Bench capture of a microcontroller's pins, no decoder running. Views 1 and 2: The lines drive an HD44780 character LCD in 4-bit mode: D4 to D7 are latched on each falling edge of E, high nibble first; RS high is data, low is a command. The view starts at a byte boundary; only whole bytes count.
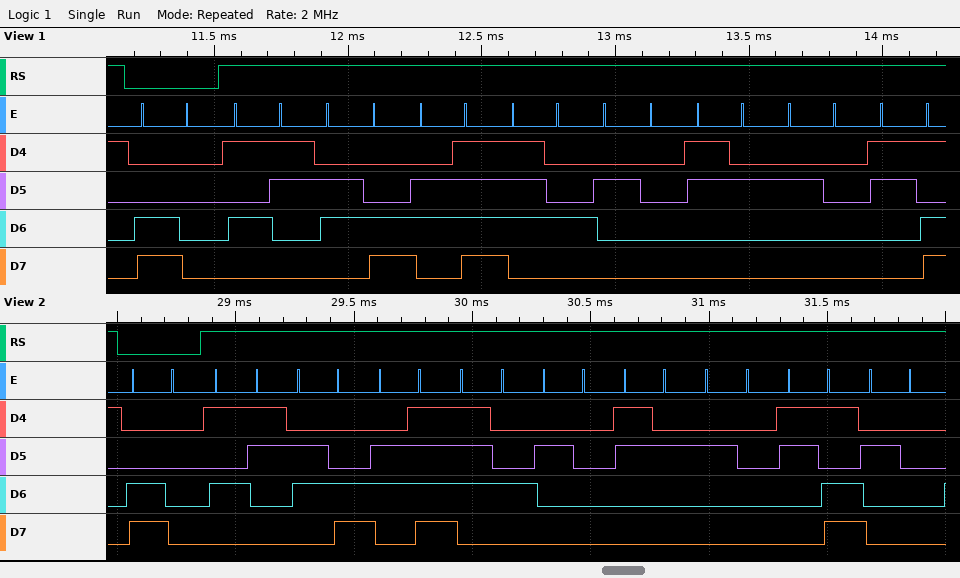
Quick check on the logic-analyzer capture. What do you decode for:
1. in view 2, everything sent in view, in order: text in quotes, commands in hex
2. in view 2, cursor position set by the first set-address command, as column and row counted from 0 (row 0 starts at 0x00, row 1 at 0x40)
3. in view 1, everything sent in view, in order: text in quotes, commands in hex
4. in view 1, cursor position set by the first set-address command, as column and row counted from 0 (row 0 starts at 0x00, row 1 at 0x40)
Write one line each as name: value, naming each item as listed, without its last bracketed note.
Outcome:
in view 2, everything sent in view, in order: text in quotes, commands in hex: 0xC0 "Slot 2 = "
in view 2, cursor position set by the first set-address command, as column and row counted from 0: column 0, row 1
in view 1, everything sent in view, in order: text in quotes, commands in hex: 0xC0 "Slot 2 ="
in view 1, cursor position set by the first set-address command, as column and row counted from 0: column 0, row 1
